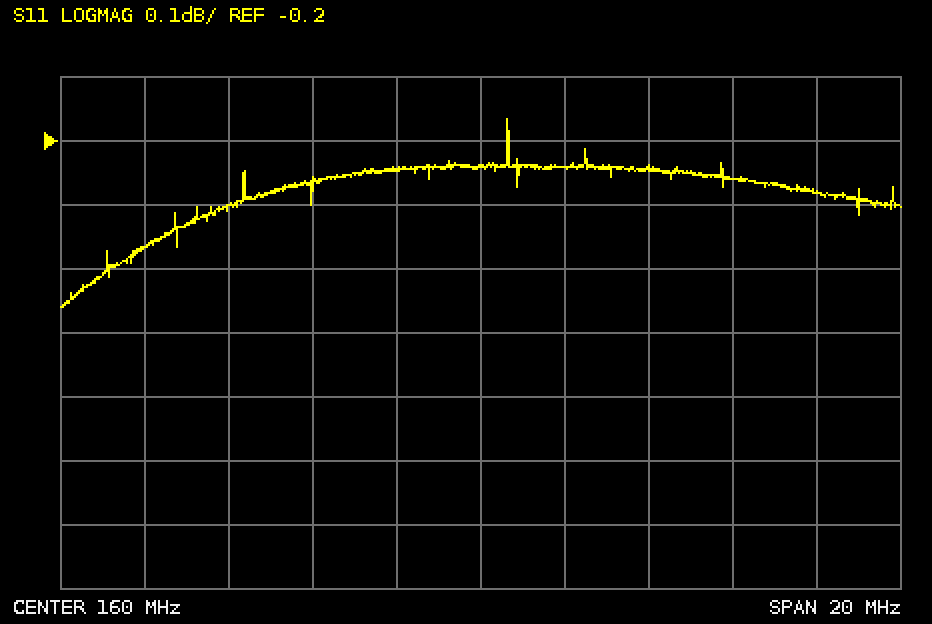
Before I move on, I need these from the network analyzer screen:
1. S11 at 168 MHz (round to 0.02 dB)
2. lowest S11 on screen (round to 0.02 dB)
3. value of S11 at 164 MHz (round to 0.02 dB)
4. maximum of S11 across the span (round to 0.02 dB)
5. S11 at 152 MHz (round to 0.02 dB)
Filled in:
-0.28 dB
-0.46 dB
-0.24 dB
-0.16 dB
-0.36 dB
